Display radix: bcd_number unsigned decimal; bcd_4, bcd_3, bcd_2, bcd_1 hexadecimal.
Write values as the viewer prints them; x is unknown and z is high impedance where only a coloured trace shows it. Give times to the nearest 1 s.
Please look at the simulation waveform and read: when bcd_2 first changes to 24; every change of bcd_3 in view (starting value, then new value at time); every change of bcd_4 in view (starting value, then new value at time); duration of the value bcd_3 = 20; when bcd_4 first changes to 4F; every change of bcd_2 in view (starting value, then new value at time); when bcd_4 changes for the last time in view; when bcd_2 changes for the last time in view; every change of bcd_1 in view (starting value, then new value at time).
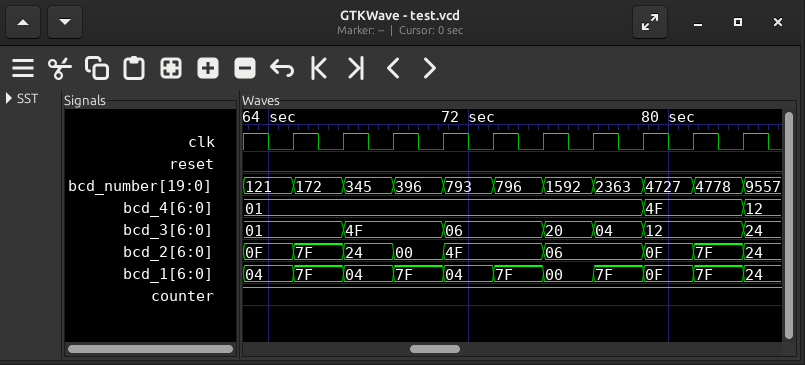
67 s
01, 4F at 67 s, 06 at 71 s, 20 at 75 s, 04 at 77 s, 12 at 79 s, 24 at 83 s
01, 4F at 79 s, 12 at 83 s
2 s
79 s
0F, 7F at 65 s, 24 at 67 s, 00 at 69 s, 4F at 71 s, 06 at 75 s, 0F at 79 s, 7F at 81 s, 24 at 83 s
83 s
83 s
04, 7F at 65 s, 04 at 67 s, 7F at 69 s, 04 at 71 s, 7F at 73 s, 00 at 75 s, 7F at 77 s, 0F at 79 s, 7F at 81 s, 24 at 83 s
